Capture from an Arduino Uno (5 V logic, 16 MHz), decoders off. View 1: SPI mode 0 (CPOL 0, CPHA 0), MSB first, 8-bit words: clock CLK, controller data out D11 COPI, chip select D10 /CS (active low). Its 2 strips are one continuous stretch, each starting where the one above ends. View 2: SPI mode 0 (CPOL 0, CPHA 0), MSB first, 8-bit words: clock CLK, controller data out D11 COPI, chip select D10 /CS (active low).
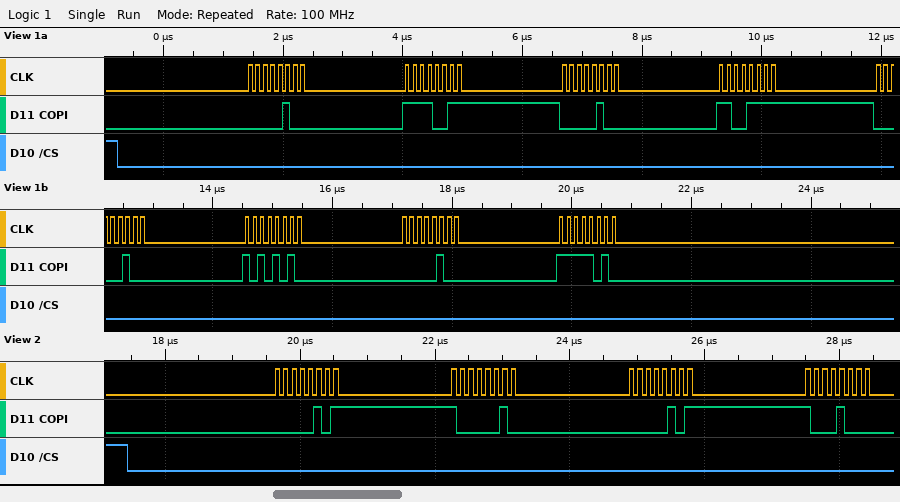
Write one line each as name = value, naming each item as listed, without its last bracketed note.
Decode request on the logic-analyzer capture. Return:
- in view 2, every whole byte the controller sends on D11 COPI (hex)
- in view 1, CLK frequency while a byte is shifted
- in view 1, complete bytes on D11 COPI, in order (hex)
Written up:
in view 2, every whole byte the controller sends on D11 COPI = 05 82 05 88
in view 1, CLK frequency while a byte is shifted = 8 MHz
in view 1, complete bytes on D11 COPI, in order = 04 F3 04 CF 04 AA 04 FA
